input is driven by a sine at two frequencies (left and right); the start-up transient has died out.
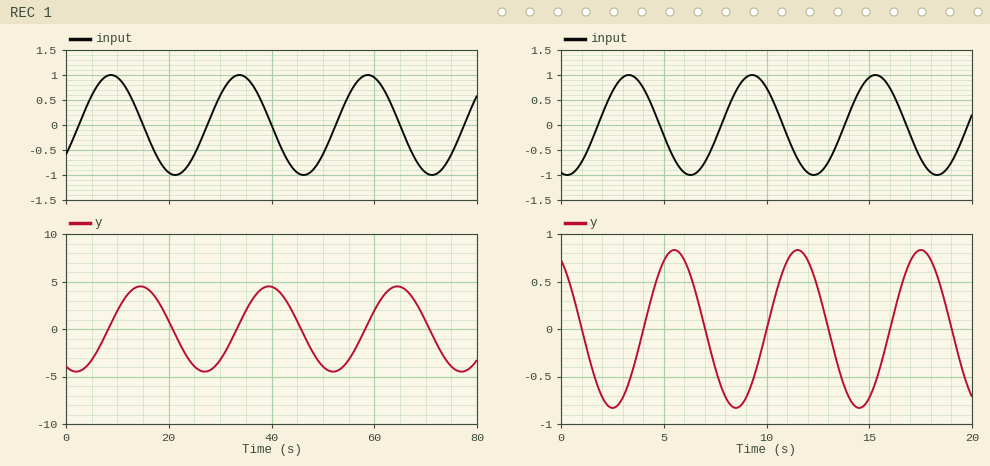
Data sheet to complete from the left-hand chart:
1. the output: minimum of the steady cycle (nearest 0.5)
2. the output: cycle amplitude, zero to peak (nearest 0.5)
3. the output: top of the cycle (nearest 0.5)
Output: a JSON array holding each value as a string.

["-4.5", "4.5", "4.5"]
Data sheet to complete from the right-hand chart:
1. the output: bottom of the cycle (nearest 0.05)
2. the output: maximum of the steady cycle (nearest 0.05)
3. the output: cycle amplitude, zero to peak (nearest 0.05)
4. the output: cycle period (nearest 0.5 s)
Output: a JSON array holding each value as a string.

["-0.85", "0.85", "0.85", "6.0 s"]
